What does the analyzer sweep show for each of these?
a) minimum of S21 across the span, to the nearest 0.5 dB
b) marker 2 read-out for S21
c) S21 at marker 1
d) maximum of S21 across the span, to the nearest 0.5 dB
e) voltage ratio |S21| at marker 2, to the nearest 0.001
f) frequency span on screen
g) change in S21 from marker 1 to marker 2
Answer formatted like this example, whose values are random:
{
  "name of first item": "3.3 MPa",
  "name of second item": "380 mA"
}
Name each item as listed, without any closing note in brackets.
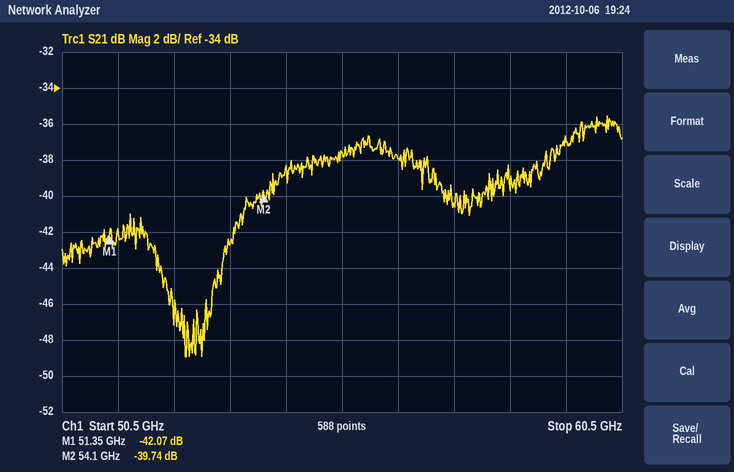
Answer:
{
  "minimum of S21 across the span, to the nearest 0.5 dB": "-49.0 dB",
  "marker 2 read-out for S21": "-39.74 dB",
  "S21 at marker 1": "-42.07 dB",
  "maximum of S21 across the span, to the nearest 0.5 dB": "-35.5 dB",
  "voltage ratio |S21| at marker 2, to the nearest 0.001": "0.010",
  "frequency span on screen": "10 GHz",
  "change in S21 from marker 1 to marker 2": "2.33 dB"
}
